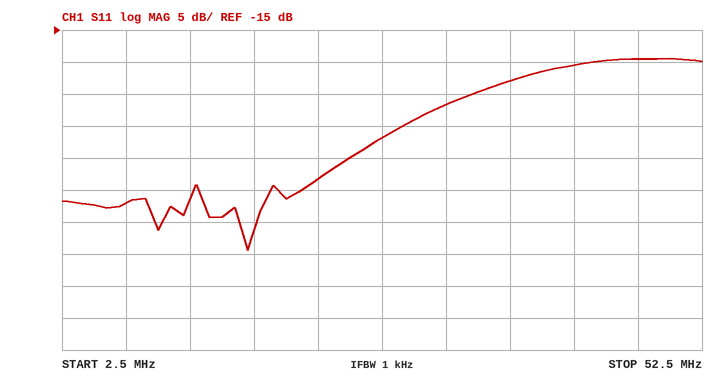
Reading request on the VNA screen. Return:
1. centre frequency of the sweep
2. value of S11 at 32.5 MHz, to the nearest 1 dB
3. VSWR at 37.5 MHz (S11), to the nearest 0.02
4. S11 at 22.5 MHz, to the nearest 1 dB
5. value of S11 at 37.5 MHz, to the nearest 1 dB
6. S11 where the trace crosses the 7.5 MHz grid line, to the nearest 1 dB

27.5 MHz
-27 dB
1.16
-38 dB
-23 dB
-42 dB
